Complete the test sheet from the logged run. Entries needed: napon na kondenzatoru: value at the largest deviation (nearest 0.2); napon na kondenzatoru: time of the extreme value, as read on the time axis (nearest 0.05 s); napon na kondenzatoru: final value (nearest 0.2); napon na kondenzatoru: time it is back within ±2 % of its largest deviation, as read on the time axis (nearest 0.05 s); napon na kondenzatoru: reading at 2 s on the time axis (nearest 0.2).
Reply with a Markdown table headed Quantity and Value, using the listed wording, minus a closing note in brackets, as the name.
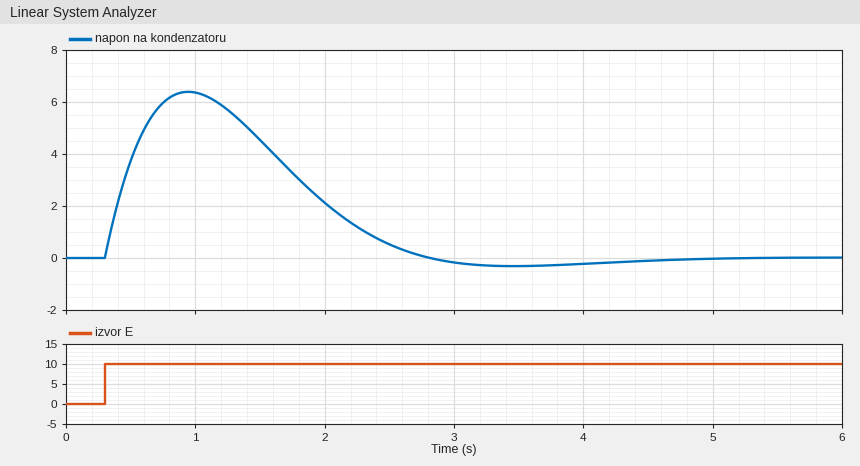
| Quantity | Value |
|---|---|
| napon na kondenzatoru: value at the largest deviation | 6.4 |
| napon na kondenzatoru: time of the extreme value, as read on the time axis | 0.95 s |
| napon na kondenzatoru: final value | 0.0 |
| napon na kondenzatoru: time it is back within ±2 % of its largest deviation, as read on the time axis | 4.40 s |
| napon na kondenzatoru: reading at 2 s on the time axis | 2.2 |
